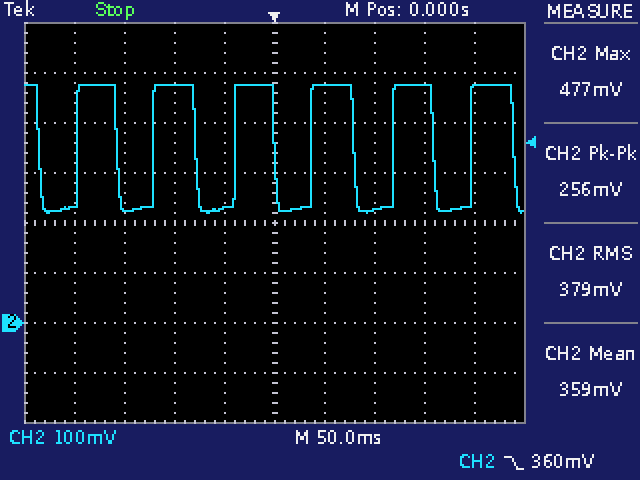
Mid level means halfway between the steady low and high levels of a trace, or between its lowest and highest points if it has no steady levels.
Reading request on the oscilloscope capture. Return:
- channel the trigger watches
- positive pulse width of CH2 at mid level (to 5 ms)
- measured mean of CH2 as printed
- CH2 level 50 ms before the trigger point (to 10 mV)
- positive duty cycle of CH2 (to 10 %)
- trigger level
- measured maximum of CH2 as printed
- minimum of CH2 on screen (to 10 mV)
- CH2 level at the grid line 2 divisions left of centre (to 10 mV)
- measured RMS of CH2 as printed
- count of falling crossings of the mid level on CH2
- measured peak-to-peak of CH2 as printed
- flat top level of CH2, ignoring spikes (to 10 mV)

CH2
40 ms
359 mV
230 mV
50 %
360 mV
477 mV
220 mV
480 mV
379 mV
7
256 mV
480 mV
